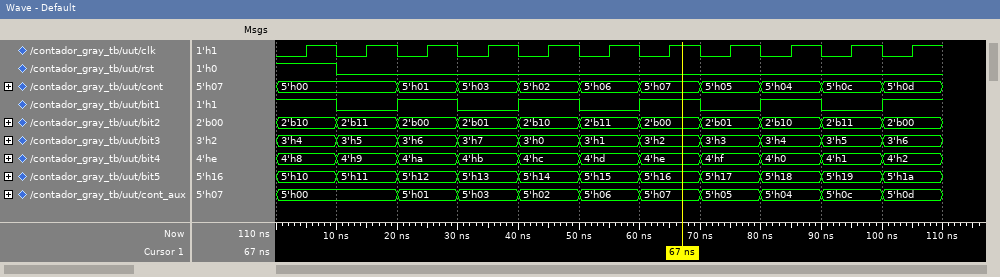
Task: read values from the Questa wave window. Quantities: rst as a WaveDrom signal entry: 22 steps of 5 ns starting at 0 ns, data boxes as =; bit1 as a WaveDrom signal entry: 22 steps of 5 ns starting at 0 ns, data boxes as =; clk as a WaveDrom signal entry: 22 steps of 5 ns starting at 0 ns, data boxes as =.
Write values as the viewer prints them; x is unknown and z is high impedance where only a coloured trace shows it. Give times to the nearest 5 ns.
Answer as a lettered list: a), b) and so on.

a) {name: 'rst', wave: '1.0...................'}
b) {name: 'bit1', wave: '1.0.1.0.1.0.1.0.1.0.1.'}
c) {name: 'clk', wave: '0101010101010101010101'}
